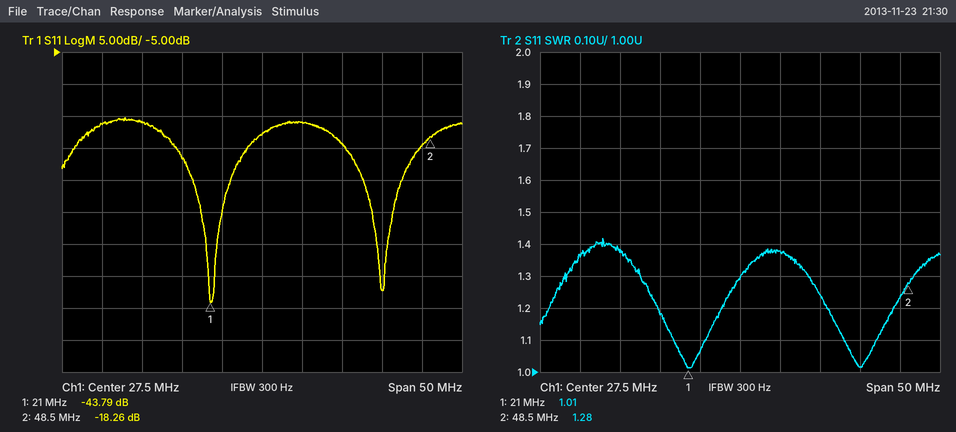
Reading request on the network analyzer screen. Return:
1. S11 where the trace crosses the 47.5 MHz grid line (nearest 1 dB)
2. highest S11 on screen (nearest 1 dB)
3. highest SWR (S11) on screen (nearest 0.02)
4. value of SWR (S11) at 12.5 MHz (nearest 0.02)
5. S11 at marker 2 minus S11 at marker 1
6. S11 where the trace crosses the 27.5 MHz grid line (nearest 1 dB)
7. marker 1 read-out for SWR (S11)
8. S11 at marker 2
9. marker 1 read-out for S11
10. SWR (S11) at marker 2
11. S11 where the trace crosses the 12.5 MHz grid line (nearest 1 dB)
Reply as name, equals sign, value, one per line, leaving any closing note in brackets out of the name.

S11 where the trace crosses the 47.5 MHz grid line = -20 dB
highest S11 on screen = -15 dB
highest SWR (S11) on screen = 1.42
value of SWR (S11) at 12.5 MHz = 1.38
S11 at marker 2 minus S11 at marker 1 = 25.53 dB
S11 where the trace crosses the 27.5 MHz grid line = -18 dB
marker 1 read-out for SWR = 1.01
S11 at marker 2 = -18.26 dB
marker 1 read-out for S11 = -43.79 dB
SWR (S11) at marker 2 = 1.28
S11 where the trace crosses the 12.5 MHz grid line = -16 dB
